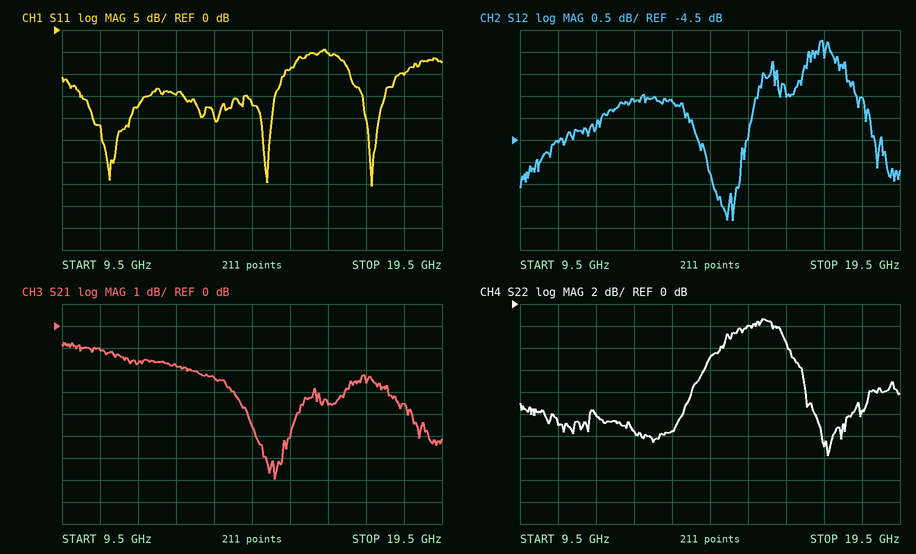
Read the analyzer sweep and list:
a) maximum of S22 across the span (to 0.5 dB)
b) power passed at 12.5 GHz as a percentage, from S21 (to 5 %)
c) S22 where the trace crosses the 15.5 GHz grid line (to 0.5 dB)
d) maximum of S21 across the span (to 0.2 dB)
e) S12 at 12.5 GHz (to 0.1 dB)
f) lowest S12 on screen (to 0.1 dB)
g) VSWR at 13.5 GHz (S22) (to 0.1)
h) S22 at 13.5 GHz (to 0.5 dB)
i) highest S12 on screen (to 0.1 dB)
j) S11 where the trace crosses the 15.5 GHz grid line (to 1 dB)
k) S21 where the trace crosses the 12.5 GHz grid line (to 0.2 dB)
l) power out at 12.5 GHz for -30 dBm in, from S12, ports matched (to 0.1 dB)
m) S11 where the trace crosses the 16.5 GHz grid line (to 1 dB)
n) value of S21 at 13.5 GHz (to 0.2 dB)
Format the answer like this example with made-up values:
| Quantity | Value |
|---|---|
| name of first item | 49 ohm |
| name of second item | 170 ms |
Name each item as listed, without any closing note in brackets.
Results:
| Quantity | Value |
|---|---|
| maximum of S22 across the span | -1.5 dB |
| power passed at 12.5 GHz as a percentage, from S21 | 65 % |
| S22 where the trace crosses the 15.5 GHz grid line | -2.0 dB |
| maximum of S21 across the span | -0.8 dB |
| S12 at 12.5 GHz | -3.6 dB |
| lowest S12 on screen | -6.3 dB |
| VSWR at 13.5 GHz (S22) | 1.7 |
| S22 at 13.5 GHz | -11.5 dB |
| highest S12 on screen | -2.2 dB |
| S11 where the trace crosses the 15.5 GHz grid line | -9 dB |
| S21 where the trace crosses the 12.5 GHz grid line | -1.8 dB |
| power out at 12.5 GHz for -30 dBm in, from S12, ports matched | -33.6 dBm |
| S11 where the trace crosses the 16.5 GHz grid line | -5 dB |
| value of S21 at 13.5 GHz | -2.4 dB |
